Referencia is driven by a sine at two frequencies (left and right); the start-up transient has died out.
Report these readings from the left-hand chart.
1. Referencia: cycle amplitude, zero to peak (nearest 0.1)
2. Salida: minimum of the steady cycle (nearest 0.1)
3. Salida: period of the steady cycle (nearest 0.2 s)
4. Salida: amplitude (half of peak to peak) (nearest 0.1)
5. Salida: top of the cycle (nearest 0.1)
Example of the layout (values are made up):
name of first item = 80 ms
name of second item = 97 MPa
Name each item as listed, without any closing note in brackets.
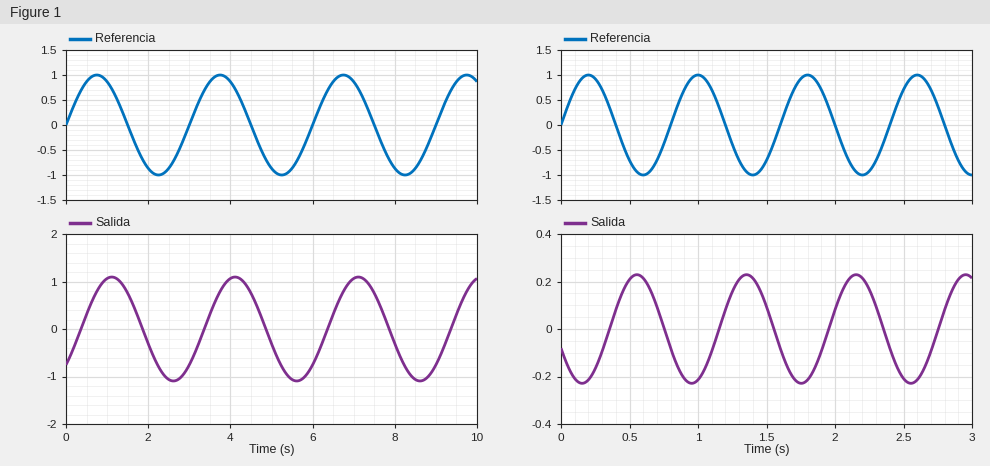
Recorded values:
Referencia: cycle amplitude, zero to peak = 1.0
Salida: minimum of the steady cycle = -1.1
Salida: period of the steady cycle = 3.0 s
Salida: amplitude (half of peak to peak) = 1.1
Salida: top of the cycle = 1.1
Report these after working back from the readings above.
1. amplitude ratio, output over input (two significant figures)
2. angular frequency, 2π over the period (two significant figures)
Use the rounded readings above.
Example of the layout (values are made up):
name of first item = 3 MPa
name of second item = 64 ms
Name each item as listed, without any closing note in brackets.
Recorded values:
amplitude ratio, output over input = 1.1
angular frequency, 2π over the period = 2.1 rad/s
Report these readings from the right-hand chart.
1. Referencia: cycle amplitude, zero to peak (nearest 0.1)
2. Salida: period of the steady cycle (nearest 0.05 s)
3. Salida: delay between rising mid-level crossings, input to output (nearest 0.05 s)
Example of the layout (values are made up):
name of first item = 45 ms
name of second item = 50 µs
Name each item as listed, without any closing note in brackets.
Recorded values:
Referencia: cycle amplitude, zero to peak = 1.0
Salida: period of the steady cycle = 0.80 s
Salida: delay between rising mid-level crossings, input to output = 0.35 s
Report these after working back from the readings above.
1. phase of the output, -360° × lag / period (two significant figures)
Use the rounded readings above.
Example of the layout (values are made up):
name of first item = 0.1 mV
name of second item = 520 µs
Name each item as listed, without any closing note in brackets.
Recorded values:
phase of the output, -360° × lag / period = -160°
